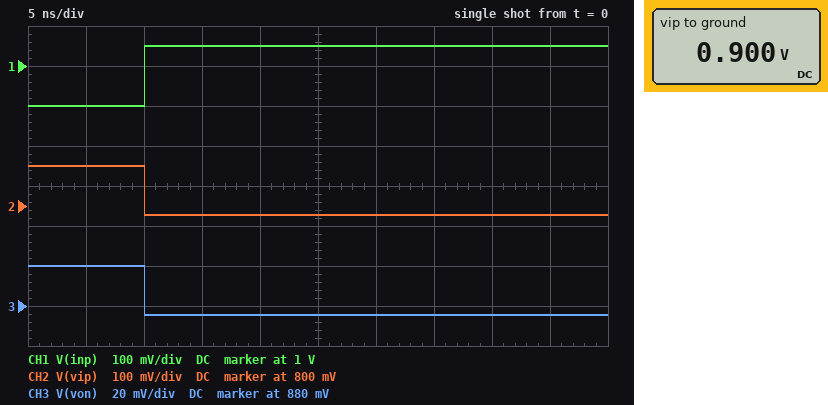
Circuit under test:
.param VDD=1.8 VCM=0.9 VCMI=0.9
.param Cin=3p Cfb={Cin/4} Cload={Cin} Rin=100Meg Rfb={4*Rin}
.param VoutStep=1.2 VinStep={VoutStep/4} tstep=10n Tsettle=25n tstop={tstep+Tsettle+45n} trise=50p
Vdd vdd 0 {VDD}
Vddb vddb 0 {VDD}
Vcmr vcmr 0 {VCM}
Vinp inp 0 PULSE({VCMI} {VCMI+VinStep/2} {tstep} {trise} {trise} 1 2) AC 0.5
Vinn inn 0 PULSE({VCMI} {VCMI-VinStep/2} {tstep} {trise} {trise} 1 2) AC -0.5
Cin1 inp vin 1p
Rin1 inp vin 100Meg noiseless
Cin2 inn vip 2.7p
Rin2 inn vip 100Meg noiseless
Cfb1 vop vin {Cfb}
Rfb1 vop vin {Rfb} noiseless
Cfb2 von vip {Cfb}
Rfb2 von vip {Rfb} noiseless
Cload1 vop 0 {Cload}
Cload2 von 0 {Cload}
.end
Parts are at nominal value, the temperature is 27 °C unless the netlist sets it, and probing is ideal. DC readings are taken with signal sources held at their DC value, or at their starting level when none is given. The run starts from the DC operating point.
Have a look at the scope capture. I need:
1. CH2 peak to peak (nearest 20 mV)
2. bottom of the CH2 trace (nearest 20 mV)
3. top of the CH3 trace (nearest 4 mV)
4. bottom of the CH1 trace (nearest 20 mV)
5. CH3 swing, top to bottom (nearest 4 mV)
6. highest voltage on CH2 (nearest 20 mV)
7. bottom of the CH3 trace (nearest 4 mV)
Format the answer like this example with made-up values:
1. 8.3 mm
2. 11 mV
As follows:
1. 120 mV
2. 780 mV
3. 900 mV
4. 900 mV
5. 24 mV
6. 900 mV
7. 876 mV
